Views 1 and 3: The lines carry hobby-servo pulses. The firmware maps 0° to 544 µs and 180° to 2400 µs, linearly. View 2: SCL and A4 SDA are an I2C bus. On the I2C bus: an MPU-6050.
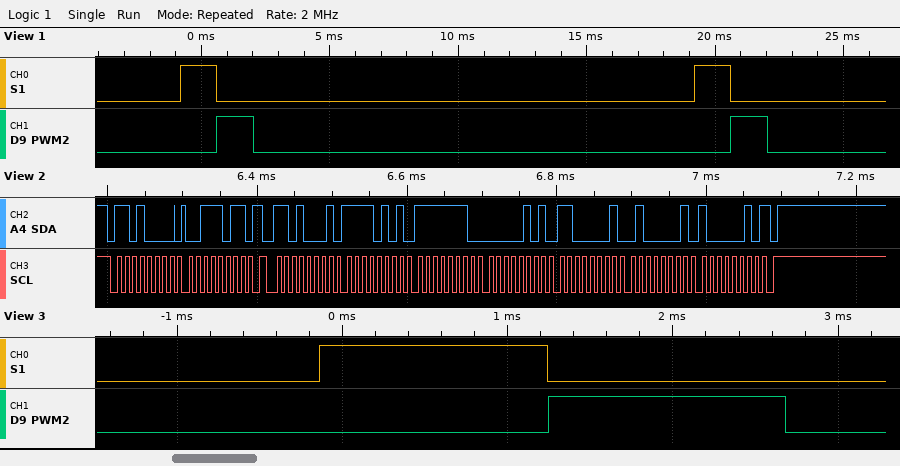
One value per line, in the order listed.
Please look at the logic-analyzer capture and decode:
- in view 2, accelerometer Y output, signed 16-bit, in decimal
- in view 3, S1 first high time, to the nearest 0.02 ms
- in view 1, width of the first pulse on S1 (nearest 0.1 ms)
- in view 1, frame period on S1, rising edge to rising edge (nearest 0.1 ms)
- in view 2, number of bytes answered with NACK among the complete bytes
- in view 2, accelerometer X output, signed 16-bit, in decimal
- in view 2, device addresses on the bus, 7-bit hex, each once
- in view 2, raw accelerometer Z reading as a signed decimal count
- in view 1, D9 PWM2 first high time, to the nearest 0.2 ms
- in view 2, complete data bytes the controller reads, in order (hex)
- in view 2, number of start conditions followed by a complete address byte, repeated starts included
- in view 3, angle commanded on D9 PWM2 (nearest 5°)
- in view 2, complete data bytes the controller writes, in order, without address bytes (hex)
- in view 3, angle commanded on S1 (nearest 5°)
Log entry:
1473
1.38 ms
1.4 ms
20.0 ms
1
-2562
0x68
16770
1.4 ms
F5 FE 05 C1 41 82
2
85°
3B
80°
